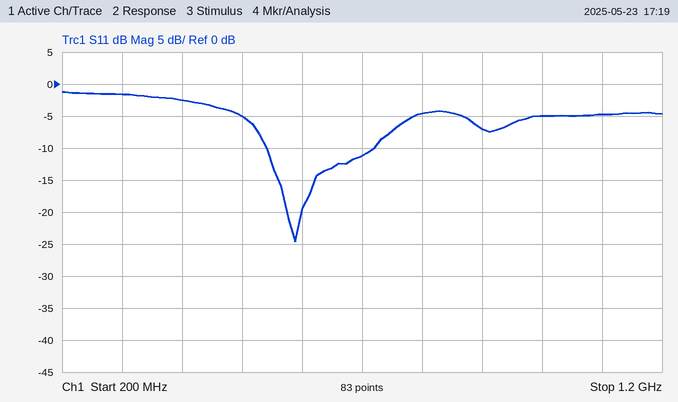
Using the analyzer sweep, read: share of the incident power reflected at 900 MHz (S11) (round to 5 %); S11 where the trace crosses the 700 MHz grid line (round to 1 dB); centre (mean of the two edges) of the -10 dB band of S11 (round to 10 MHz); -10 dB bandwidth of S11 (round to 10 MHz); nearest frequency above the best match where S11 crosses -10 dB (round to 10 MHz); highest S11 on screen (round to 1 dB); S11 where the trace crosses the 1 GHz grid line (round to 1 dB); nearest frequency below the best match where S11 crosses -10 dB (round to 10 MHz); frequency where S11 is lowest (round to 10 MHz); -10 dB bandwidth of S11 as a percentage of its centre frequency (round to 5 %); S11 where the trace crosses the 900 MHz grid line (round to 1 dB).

20 %
-11 dB
630 MHz
180 MHz
720 MHz
-1 dB
-5 dB
540 MHz
590 MHz
30 %
-7 dB
